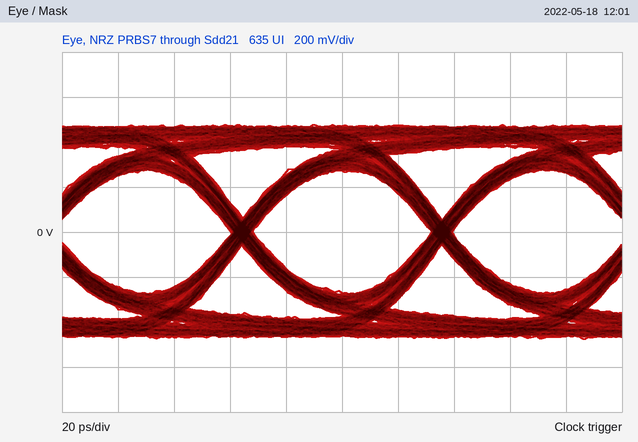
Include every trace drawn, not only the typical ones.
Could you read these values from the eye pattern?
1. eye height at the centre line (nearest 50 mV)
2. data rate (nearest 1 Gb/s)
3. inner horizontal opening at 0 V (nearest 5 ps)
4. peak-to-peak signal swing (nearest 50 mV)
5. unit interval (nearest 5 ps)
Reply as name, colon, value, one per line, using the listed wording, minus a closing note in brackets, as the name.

eye height at the centre line: 550 mV
data rate: 14 Gb/s
inner horizontal opening at 0 V: 65 ps
peak-to-peak signal swing: 950 mV
unit interval: 70 ps
